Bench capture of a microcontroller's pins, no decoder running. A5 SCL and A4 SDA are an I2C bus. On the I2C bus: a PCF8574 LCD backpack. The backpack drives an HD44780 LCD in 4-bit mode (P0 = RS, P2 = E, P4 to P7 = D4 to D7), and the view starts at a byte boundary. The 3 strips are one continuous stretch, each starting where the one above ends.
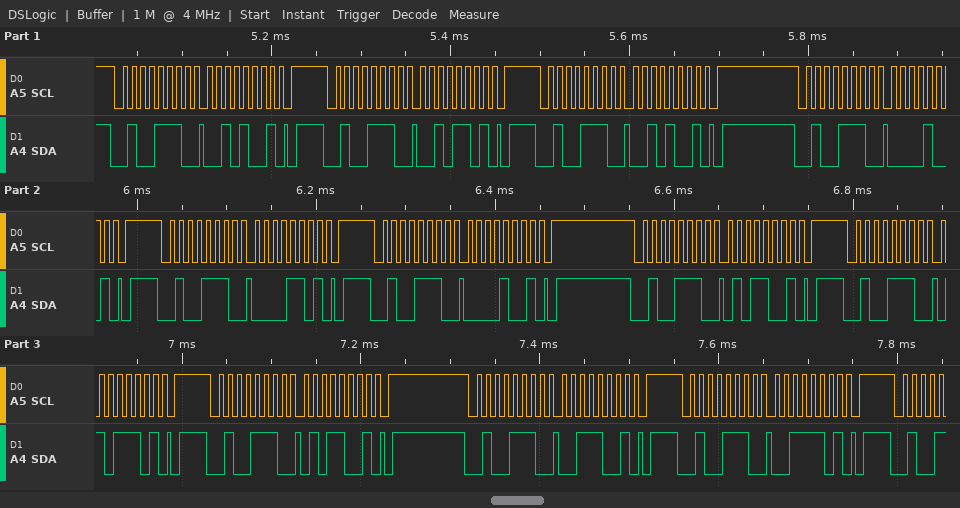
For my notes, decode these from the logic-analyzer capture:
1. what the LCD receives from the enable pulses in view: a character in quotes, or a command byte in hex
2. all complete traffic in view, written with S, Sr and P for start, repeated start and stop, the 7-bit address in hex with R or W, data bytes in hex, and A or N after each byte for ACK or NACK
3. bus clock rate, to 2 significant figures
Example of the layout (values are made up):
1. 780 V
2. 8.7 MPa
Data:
1. ' '
2. S 27W A 29 A P S 27W A 2D A P S 27W A 29 A P S 27W A 09 A P S 27W A 0D A P S 27W A 09 A P S 27W A 59 A P S 27W A 5D A P S 27W A 59 A P S 27W A 39 A P S 27W A 3D A P
3. 100 kHz
